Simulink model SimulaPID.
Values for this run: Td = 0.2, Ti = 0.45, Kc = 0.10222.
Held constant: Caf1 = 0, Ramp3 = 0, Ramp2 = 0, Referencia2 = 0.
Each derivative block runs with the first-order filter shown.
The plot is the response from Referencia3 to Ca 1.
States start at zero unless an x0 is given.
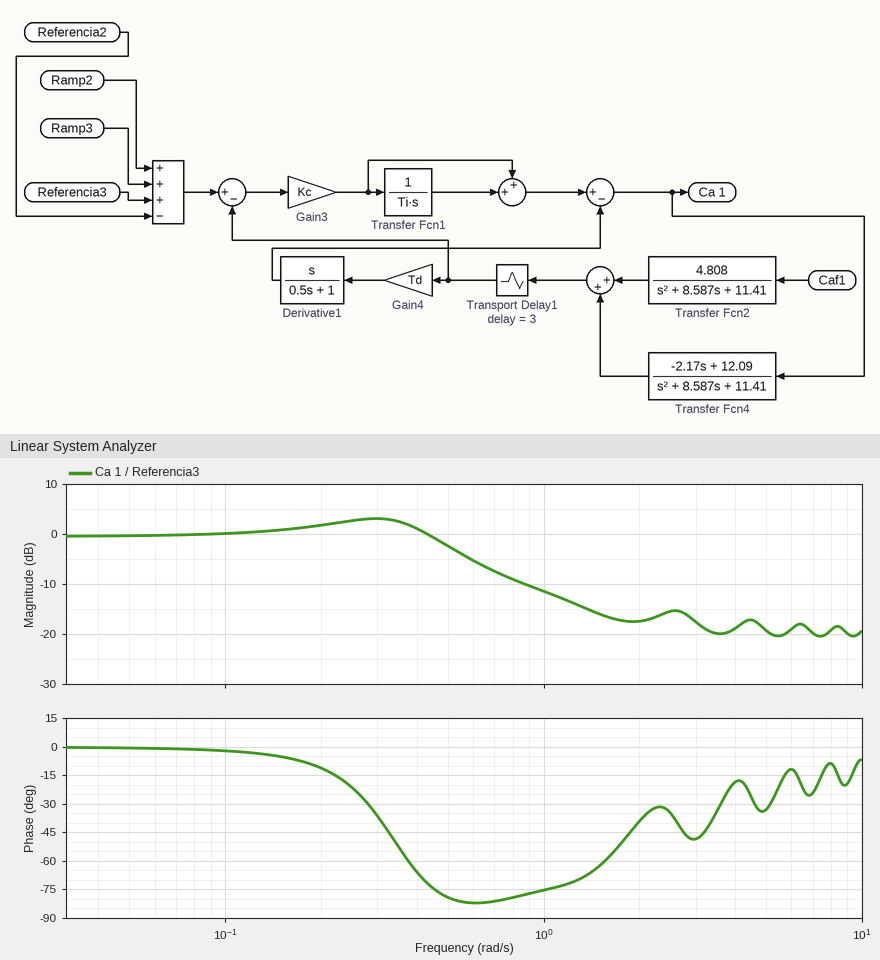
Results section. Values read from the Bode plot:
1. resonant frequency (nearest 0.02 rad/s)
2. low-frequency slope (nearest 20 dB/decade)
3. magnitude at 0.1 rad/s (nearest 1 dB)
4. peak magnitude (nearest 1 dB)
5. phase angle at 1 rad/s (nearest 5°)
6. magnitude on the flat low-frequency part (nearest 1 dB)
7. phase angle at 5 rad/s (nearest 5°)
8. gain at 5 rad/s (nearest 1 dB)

0.30 rad/s
0 dB/decade
0 dB
3 dB
-75°
0 dB
-35°
-19 dB
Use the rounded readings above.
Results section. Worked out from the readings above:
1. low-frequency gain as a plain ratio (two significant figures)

1.0
